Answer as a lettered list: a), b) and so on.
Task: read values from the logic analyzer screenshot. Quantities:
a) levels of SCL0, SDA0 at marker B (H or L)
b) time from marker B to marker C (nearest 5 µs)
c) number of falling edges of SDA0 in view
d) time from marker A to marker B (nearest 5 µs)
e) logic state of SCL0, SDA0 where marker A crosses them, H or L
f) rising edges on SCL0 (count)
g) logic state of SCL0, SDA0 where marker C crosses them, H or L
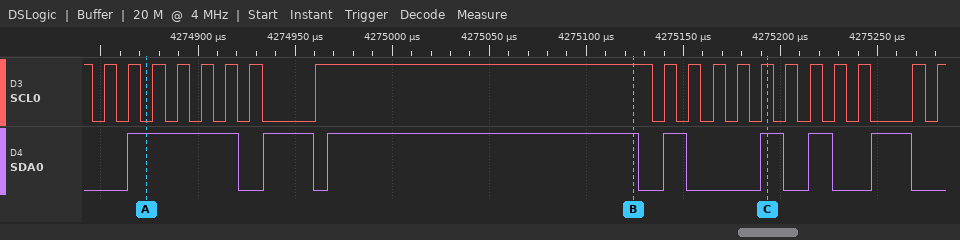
a) SCL0=H, SDA0=H
b) 70 µs
c) 7
d) 250 µs
e) SCL0=L, SDA0=H
f) 19
g) SCL0=H, SDA0=H
